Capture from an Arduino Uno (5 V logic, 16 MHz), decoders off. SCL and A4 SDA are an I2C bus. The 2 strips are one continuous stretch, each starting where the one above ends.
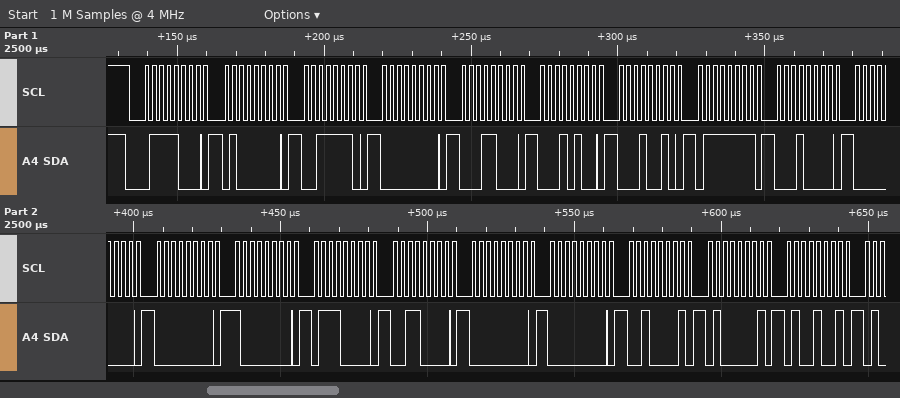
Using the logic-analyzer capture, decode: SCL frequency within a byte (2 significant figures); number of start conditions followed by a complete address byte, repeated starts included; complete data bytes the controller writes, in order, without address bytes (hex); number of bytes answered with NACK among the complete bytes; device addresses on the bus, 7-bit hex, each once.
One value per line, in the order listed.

400 kHz
1
40 3E 00 18 14 12 7F 10 00 00 80 70 30 00 00 21 41 49
0
0x3C
